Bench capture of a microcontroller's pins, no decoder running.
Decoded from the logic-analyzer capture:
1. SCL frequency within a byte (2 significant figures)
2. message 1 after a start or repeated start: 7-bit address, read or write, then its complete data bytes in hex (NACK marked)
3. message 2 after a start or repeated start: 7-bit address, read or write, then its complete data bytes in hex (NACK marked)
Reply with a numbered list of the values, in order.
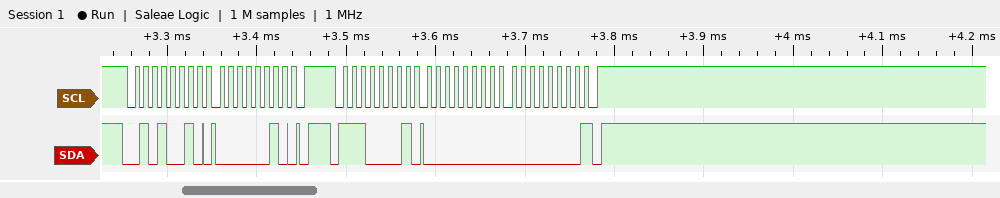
1. 100 kHz
2. 0x29 write: 02
3. 0x70 read: 00 00 NACK
